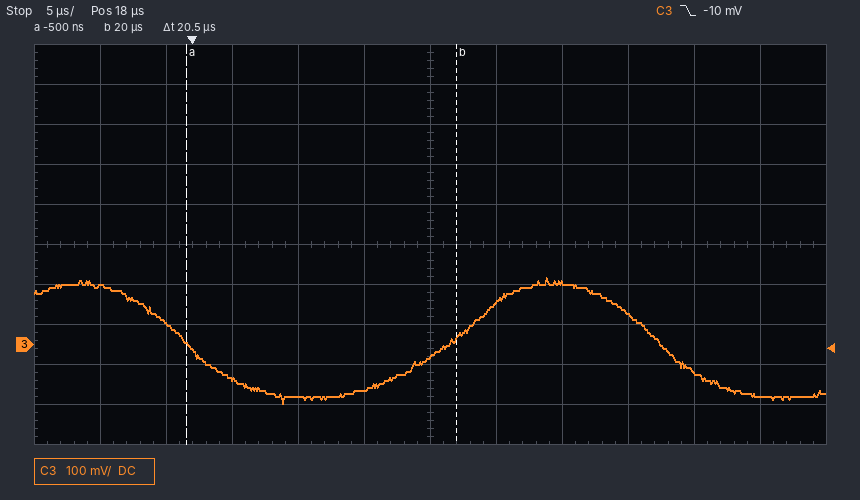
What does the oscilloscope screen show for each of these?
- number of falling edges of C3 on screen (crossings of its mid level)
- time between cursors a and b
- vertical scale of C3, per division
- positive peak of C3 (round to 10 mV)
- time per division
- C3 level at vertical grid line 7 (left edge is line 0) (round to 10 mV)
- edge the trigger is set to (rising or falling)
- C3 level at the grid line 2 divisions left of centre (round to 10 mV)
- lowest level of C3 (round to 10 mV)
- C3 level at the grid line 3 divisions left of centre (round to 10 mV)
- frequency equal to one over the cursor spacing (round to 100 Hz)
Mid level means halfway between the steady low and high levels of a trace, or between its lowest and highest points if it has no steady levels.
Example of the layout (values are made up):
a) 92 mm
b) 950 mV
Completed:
a) 2
b) 20.5 µs
c) 100 mV
d) 170 mV
e) 5 µs
f) 100 mV
g) falling
h) -130 mV
i) -150 mV
j) -90 mV
k) 48.8 kHz
